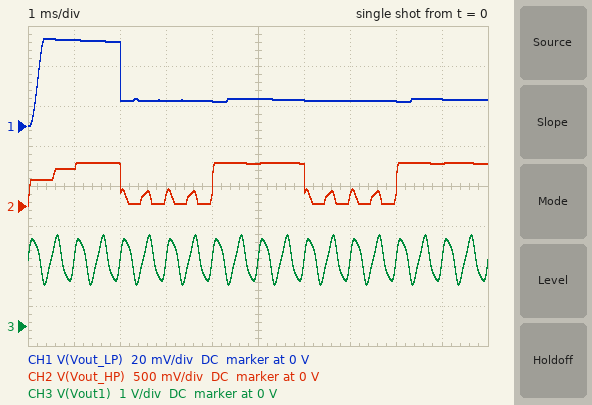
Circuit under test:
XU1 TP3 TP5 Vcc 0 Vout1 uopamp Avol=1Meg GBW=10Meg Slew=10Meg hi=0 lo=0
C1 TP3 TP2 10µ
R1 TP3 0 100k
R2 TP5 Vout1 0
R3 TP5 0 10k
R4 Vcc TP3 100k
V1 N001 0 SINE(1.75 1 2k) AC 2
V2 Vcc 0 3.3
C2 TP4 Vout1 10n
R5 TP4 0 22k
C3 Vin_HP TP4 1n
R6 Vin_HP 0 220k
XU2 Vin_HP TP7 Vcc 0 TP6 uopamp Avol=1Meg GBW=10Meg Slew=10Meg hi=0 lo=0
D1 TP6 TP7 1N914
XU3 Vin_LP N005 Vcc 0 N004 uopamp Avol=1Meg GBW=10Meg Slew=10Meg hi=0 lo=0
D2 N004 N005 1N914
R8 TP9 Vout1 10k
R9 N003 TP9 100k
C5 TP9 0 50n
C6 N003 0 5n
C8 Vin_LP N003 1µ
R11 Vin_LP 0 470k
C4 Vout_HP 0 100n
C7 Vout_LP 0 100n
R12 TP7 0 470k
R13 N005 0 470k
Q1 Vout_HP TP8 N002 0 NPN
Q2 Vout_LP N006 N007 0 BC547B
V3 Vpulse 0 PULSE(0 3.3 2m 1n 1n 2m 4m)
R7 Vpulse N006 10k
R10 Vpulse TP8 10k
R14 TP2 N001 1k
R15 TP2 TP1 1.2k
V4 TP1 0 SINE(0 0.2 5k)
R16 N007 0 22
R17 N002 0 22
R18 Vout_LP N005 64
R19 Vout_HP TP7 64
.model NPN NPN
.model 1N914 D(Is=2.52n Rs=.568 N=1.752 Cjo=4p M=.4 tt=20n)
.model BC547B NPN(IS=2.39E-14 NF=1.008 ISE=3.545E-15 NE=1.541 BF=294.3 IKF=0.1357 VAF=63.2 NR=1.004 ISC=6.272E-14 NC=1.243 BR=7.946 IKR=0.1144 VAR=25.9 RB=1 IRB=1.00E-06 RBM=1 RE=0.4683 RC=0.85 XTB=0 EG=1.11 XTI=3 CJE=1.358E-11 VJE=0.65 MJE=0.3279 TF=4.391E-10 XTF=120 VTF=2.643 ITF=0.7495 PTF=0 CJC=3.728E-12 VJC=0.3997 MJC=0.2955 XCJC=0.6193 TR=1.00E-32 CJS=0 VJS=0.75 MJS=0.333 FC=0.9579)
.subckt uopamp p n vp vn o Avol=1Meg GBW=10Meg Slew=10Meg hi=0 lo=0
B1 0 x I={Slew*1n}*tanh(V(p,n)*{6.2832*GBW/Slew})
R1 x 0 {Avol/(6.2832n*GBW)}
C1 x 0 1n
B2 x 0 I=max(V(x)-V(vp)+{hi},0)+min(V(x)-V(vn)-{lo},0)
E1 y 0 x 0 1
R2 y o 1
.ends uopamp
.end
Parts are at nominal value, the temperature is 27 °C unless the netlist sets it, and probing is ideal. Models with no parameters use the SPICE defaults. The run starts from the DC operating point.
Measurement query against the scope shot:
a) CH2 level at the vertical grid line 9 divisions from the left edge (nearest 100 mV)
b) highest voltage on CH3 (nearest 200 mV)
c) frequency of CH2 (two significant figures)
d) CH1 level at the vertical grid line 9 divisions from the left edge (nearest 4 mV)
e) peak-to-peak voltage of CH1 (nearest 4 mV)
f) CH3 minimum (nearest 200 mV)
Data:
500 mV
2.2 V
250 Hz
12 mV
44 mV
1.0 V
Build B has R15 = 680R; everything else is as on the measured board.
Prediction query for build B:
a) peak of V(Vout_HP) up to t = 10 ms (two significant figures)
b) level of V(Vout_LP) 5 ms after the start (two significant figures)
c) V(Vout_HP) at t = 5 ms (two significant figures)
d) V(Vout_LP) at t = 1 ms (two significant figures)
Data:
450 mV
12 mV
440 mV
33 mV
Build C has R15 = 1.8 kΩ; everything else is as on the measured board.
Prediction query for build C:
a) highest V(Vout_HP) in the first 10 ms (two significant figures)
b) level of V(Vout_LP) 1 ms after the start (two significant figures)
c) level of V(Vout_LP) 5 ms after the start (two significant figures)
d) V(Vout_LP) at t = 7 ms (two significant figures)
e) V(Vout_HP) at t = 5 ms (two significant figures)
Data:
610 mV
50 mV
16 mV
12 mV
590 mV
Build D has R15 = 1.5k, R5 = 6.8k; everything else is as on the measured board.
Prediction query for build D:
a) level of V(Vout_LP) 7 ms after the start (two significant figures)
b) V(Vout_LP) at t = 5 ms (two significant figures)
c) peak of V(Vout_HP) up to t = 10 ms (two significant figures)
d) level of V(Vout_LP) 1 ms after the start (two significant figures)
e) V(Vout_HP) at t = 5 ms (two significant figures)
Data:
12 mV
15 mV
420 mV
47 mV
410 mV
